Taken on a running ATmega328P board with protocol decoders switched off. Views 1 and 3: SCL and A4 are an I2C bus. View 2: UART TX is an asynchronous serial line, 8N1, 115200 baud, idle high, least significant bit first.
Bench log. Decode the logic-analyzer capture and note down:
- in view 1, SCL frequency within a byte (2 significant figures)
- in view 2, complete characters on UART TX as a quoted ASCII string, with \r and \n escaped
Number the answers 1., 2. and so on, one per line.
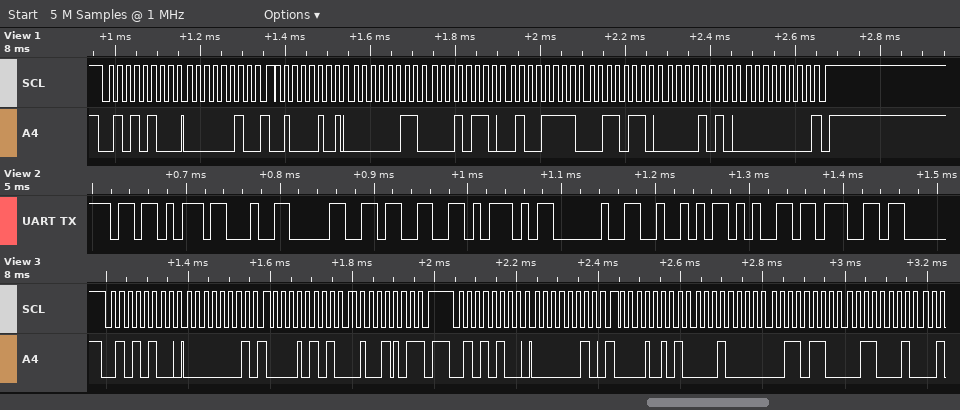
1. 50 kHz
2. "[#03] Reg"
